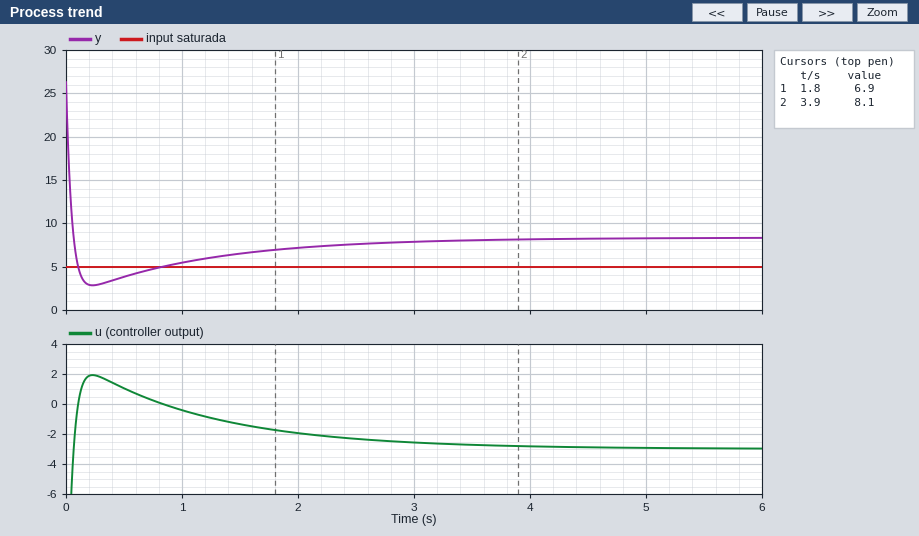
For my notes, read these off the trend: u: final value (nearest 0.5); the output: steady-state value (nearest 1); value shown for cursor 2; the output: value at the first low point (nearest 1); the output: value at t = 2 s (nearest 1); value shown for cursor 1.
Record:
-3.0
8
8.1
3
7
6.9
